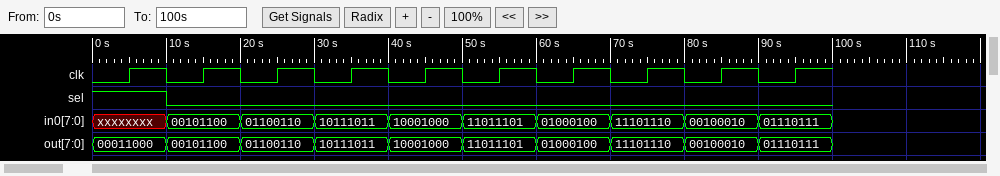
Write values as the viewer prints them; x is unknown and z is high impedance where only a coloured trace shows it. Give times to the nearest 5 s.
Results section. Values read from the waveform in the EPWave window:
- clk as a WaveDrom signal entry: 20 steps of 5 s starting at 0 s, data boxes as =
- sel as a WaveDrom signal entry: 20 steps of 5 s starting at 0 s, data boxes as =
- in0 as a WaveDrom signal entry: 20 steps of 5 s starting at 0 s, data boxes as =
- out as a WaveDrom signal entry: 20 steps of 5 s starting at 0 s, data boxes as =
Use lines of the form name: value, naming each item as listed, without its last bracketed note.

clk as a WaveDrom signal entry: 20 steps of 5 s starting at 0 s, data boxes as =: {name: 'clk', wave: '01010101010101010101'}
sel as a WaveDrom signal entry: 20 steps of 5 s starting at 0 s, data boxes as =: {name: 'sel', wave: '1.0.................'}
in0 as a WaveDrom signal entry: 20 steps of 5 s starting at 0 s, data boxes as =: {name: 'in0', wave: 'x.=.=.=.=.=.=.=.=.=.', data: '00101100 01100110 10111011 10001000 11011101 01000100 11101110 00100010 01110111'}
out as a WaveDrom signal entry: 20 steps of 5 s starting at 0 s, data boxes as =: {name: 'out', wave: '=.=.=.=.=.=.=.=.=.=.', data: '00011000 00101100 01100110 10111011 10001000 11011101 01000100 11101110 00100010 01110111'}
